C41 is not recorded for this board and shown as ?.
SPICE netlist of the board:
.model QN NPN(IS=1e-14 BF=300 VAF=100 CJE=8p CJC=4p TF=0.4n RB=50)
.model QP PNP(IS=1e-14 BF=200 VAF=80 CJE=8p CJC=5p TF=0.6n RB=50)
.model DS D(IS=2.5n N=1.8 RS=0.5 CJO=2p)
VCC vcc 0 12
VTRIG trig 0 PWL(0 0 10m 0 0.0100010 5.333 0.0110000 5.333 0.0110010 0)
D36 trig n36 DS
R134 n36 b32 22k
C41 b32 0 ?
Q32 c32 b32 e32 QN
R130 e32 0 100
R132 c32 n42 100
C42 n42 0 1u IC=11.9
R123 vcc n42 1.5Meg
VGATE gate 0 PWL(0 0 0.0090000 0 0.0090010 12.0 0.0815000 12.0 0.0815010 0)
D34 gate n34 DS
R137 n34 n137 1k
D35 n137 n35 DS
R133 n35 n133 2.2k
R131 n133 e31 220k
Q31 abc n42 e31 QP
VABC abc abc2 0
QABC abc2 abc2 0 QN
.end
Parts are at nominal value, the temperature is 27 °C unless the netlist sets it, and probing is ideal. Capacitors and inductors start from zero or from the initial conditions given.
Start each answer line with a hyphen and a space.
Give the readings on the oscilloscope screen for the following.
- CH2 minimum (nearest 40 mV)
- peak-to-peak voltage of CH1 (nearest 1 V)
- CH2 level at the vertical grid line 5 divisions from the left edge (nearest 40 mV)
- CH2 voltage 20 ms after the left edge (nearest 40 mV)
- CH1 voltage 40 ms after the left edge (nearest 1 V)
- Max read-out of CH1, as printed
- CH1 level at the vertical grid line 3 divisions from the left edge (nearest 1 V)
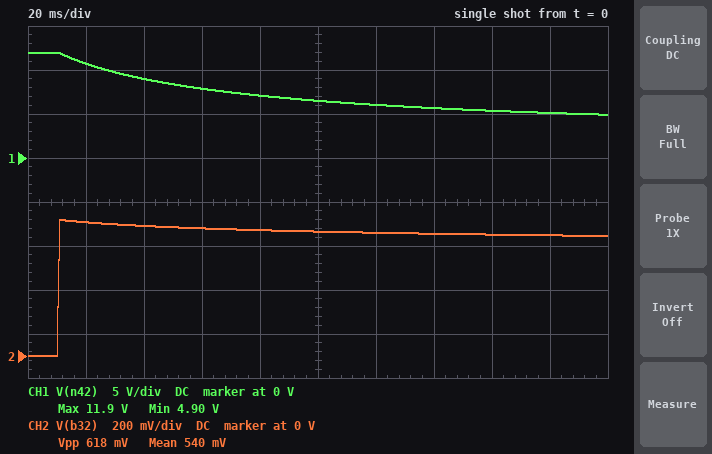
- 0 V
- 7 V
- 560 mV
- 600 mV
- 9 V
- 11.9 V
- 8 V
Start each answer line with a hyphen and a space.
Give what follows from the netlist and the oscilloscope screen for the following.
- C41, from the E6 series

- 330 nF
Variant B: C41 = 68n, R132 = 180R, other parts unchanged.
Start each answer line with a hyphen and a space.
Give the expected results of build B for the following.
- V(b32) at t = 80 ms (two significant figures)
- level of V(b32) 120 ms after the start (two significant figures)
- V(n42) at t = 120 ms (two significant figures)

- 500 mV
- 490 mV
- 650 mV
